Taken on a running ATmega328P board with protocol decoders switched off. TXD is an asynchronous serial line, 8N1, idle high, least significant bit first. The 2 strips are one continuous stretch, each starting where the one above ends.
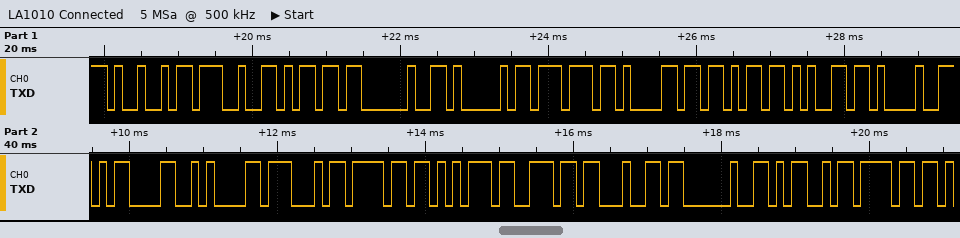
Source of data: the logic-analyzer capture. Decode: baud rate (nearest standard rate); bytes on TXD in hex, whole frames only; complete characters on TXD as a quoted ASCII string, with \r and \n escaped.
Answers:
9600 baud
0x49 0x27 0x6D 0x20 0x41 0x77 0x61 0x6B 0x65 0x21 0x0D 0x0A 0x47 0x6F 0x75 0x6E 0x64 0x20 0x4D 0x6F
"I'm Awake!\r\nGound Mo"
